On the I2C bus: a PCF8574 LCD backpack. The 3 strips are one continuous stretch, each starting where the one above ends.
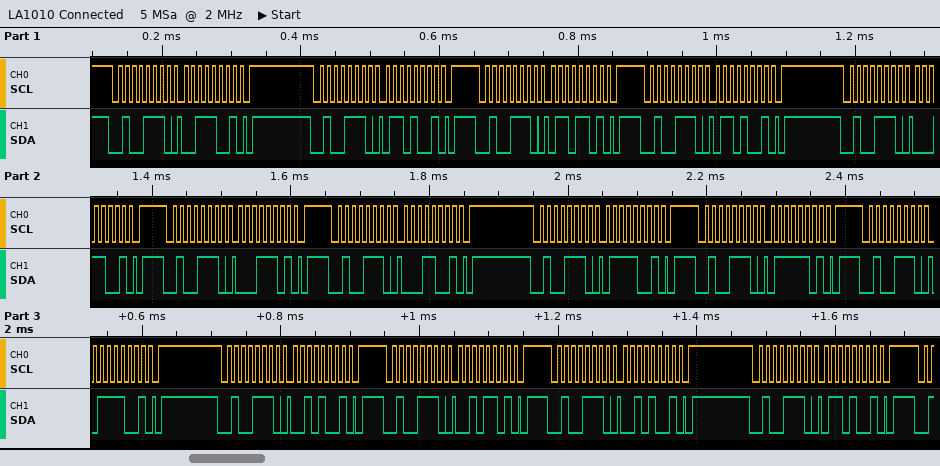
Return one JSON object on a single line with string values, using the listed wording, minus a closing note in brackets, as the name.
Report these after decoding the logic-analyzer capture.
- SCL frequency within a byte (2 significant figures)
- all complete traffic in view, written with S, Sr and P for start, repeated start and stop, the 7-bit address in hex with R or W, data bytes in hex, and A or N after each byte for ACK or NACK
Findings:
{"SCL frequency within a byte": "100 kHz", "all complete traffic in view, written with S, Sr and P for start, repeated start and stop, the 7-bit address in hex with R or W, data bytes in hex, and A or N after each byte for ACK or NACK": "S 27W A 39 A P S 27W A 69 A P S 27W A 6D A P S 27W A 69 A P S 27W A 19 A P S 27W A 1D A P S 27W A 19 A P S 27W A 79 A P S 27W A 7D A P S 27W A 79 A P S 27W A 29 A P S 27W A 2D A P S 27W A 29 A P S 27W A 69 A P"}
